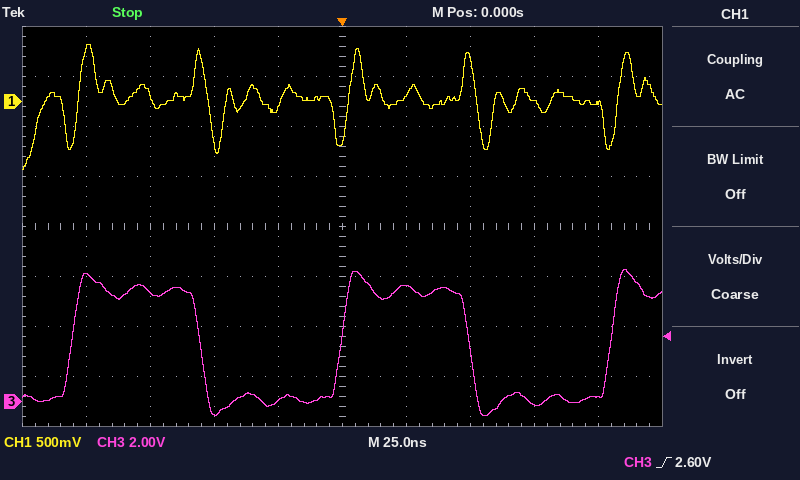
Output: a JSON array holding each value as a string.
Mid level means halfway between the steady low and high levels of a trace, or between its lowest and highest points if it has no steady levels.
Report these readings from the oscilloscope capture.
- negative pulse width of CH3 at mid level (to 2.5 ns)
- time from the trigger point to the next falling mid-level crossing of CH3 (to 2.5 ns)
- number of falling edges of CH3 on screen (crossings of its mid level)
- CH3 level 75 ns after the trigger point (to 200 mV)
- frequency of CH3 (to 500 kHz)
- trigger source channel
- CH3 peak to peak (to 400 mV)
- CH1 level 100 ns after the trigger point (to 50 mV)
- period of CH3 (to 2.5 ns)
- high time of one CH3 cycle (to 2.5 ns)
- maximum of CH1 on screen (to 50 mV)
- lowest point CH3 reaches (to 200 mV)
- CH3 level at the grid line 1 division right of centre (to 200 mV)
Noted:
["55.0 ns", "50.0 ns", "2", "-200 mV", "9.5 MHz", "CH3", "6.0 V", "0 mV", "105.0 ns", "50.0 ns", "550 mV", "-600 mV", "4.6 V"]
